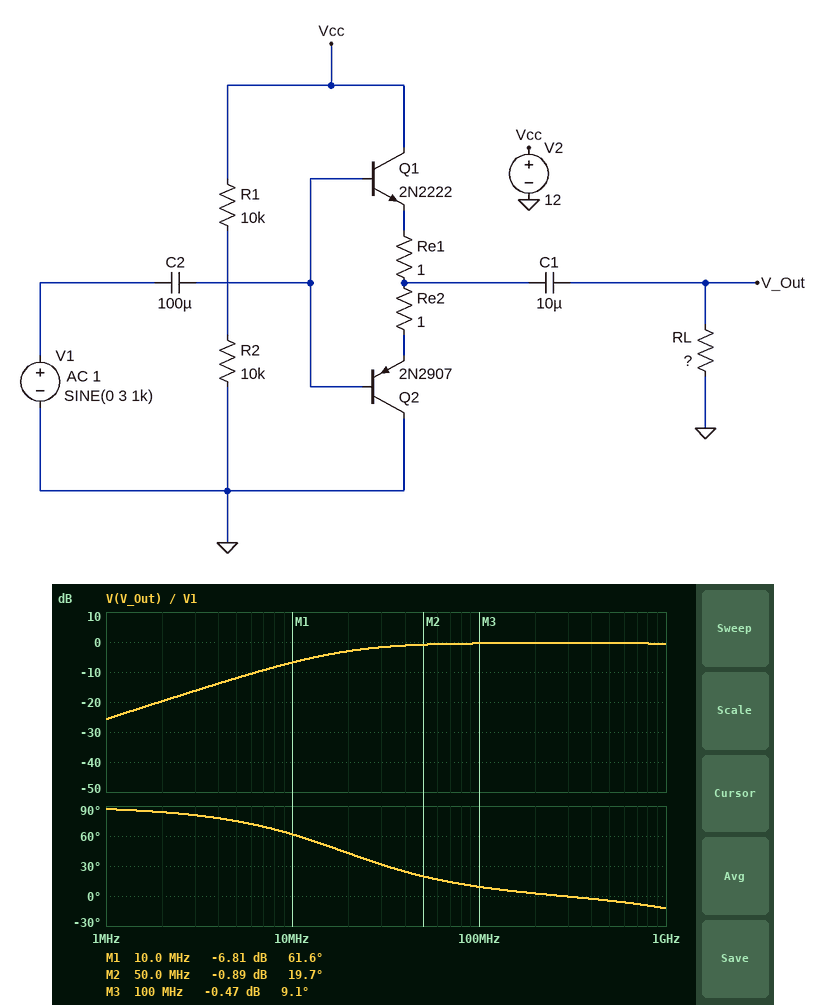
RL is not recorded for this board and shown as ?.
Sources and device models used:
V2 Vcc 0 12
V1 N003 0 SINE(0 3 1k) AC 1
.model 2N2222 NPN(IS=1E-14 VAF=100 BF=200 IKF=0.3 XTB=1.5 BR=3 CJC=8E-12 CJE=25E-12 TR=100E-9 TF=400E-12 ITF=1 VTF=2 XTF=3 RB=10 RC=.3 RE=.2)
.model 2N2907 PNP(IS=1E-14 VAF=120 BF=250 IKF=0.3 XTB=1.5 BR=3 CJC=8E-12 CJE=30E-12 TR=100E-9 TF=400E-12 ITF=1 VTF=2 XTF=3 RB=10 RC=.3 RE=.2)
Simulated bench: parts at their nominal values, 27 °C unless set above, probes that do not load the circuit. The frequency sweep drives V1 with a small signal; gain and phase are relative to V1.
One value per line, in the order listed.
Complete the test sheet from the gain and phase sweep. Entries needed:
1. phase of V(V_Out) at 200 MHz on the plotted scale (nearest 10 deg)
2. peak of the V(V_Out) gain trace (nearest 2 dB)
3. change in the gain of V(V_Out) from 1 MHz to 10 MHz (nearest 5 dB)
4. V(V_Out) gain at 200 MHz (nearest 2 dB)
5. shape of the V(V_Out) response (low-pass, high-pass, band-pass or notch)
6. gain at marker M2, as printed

0 deg
0 dB
20 dB
0 dB
high-pass
-0.89 dB
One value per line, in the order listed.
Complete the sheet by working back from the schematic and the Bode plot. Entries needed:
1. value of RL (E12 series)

150 Ω
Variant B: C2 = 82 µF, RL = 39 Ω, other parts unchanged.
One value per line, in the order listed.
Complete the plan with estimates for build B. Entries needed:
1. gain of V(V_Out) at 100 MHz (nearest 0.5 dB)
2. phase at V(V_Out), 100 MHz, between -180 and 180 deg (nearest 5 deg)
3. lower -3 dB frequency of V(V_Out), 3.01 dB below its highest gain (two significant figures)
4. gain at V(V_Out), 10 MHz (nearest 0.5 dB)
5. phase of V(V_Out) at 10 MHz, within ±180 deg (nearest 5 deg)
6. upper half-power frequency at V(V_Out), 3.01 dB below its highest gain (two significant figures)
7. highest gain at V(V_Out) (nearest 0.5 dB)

-2.5 dB
30 deg
63 MHz
-17.5 dB
80 deg
4.5 GHz
-1.5 dB
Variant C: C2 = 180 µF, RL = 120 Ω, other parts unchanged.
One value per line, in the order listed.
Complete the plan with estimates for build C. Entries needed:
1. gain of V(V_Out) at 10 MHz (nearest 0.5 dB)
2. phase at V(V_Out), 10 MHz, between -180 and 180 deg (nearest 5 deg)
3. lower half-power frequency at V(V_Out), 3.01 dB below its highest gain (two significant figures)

-8.5 dB
65 deg
23 MHz
